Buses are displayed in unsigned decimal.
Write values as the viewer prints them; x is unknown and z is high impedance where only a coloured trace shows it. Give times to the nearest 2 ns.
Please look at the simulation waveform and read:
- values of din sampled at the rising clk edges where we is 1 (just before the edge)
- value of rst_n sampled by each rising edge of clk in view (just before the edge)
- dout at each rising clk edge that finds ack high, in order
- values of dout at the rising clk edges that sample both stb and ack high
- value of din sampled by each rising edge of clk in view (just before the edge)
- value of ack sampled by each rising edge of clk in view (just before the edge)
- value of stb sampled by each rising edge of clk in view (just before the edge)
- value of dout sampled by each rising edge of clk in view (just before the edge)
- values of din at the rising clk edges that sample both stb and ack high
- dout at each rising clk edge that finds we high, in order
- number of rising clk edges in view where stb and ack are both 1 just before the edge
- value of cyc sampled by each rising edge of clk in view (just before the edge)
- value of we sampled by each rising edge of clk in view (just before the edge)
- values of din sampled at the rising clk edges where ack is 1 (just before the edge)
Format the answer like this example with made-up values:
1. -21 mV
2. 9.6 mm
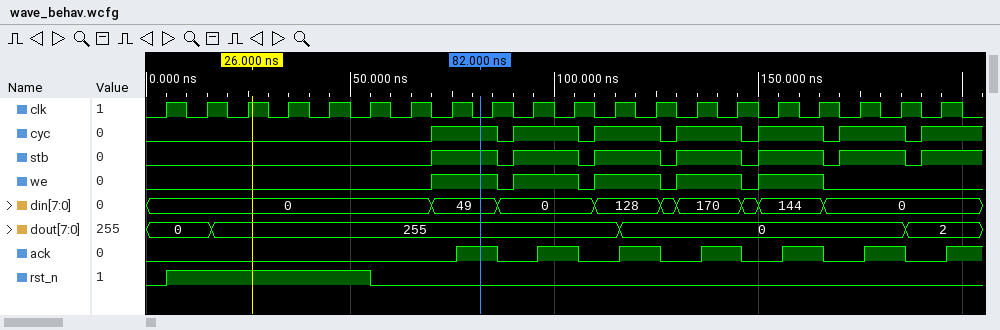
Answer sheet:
1. 49, 49, 0, 0, 128, 128, 170, 170, 144, 144
2. 0 1 1 1 1 1 0 0 0 0 0 0 0 0 0 0 0 0 0 0
3. 255, 255, 0, 0, 0, 0
4. 255, 255, 0, 0, 0, 0
5. 0, 0, 0, 0, 0, 0, 0, 49, 49, 0, 0, 128, 128, 170, 170, 144, 144, 0, 0, 0
6. 0 0 0 0 0 0 0 0 1 0 1 0 1 0 1 0 1 0 1 0
7. 0 0 0 0 0 0 0 1 1 1 1 1 1 1 1 1 1 1 1 1
8. 0, 0, 255, 255, 255, 255, 255, 255, 255, 255, 255, 255, 0, 0, 0, 0, 0, 0, 0, 2
9. 49, 0, 128, 170, 144, 0
10. 255, 255, 255, 255, 255, 0, 0, 0, 0, 0
11. 6
12. 0 0 0 0 0 0 0 1 1 1 1 1 1 1 1 1 1 1 1 1
13. 0 0 0 0 0 0 0 1 1 1 1 1 1 1 1 1 1 0 0 0
14. 49, 0, 128, 170, 144, 0
